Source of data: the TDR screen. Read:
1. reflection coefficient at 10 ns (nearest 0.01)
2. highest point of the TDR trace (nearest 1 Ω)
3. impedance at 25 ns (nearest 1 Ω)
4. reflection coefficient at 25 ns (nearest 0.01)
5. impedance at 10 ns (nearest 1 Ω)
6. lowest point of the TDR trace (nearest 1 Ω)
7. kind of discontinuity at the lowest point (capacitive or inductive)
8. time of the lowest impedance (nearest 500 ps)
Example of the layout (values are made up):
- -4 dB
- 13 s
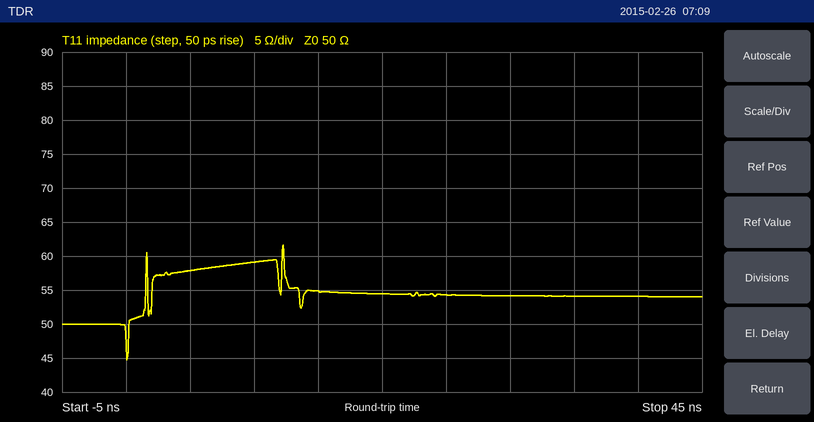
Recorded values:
- +0.08
- 62 Ω
- 54 Ω
- +0.04
- 59 Ω
- 45 Ω
- capacitive
- 0.0 ns
